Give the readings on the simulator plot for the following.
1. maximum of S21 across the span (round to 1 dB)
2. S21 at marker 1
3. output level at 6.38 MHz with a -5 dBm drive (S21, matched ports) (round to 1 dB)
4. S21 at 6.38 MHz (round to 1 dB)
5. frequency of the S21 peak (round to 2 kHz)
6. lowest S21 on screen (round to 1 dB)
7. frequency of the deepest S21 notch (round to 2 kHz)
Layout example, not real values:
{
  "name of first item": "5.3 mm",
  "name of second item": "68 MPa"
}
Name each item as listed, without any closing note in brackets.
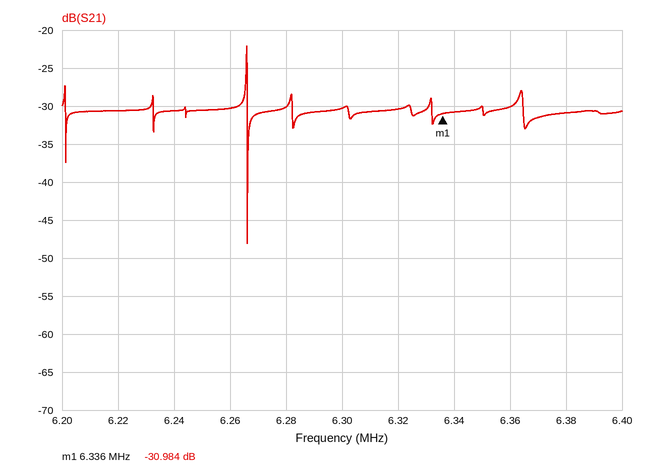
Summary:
{
  "maximum of S21 across the span": "-22 dB",
  "S21 at marker 1": "-30.984 dB",
  "output level at 6.38 MHz with a -5 dBm drive (S21, matched ports)": "-36 dBm",
  "S21 at 6.38 MHz": "-31 dB",
  "frequency of the S21 peak": "6.266 MHz",
  "lowest S21 on screen": "-48 dB",
  "frequency of the deepest S21 notch": "6.266 MHz"
}
